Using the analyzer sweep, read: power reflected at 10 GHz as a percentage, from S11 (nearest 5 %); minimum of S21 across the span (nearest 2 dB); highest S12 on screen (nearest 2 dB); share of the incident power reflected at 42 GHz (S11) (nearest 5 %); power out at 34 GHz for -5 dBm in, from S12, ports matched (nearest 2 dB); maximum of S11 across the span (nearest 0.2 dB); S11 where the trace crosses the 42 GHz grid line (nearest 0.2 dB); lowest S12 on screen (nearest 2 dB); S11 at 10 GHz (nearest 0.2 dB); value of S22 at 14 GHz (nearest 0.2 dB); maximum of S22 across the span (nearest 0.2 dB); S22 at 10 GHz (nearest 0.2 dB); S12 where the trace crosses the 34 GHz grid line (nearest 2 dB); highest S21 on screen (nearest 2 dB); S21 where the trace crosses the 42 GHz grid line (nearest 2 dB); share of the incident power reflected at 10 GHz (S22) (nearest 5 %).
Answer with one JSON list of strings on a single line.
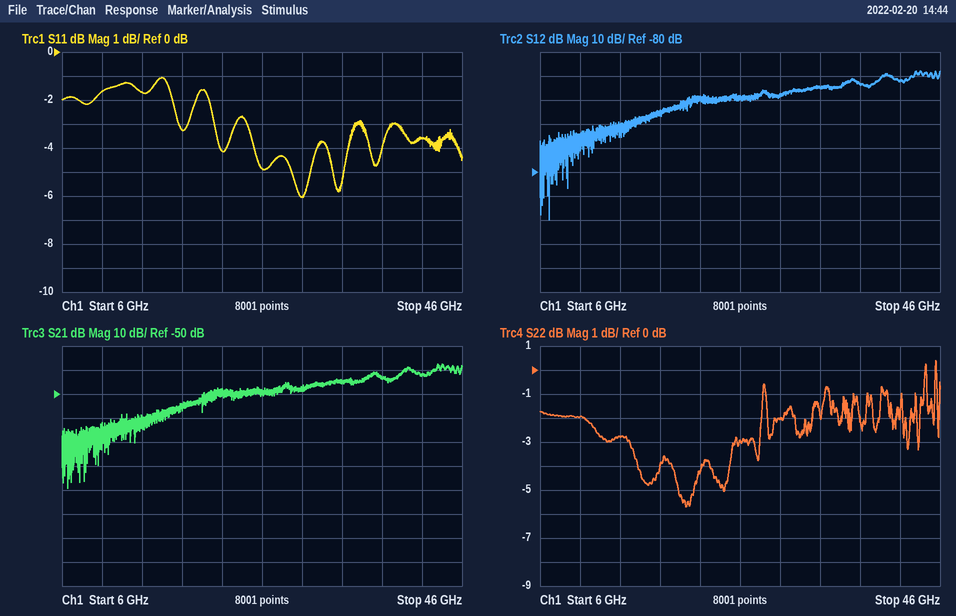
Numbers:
["70 %", "-90 dB", "-38 dB", "45 %", "-50 dBm", "-1.0 dB", "-3.6 dB", "-100 dB", "-1.6 dB", "-2.8 dB", "0.4 dB", "-2.0 dB", "-44 dB", "-38 dB", "-42 dB", "65 %"]
